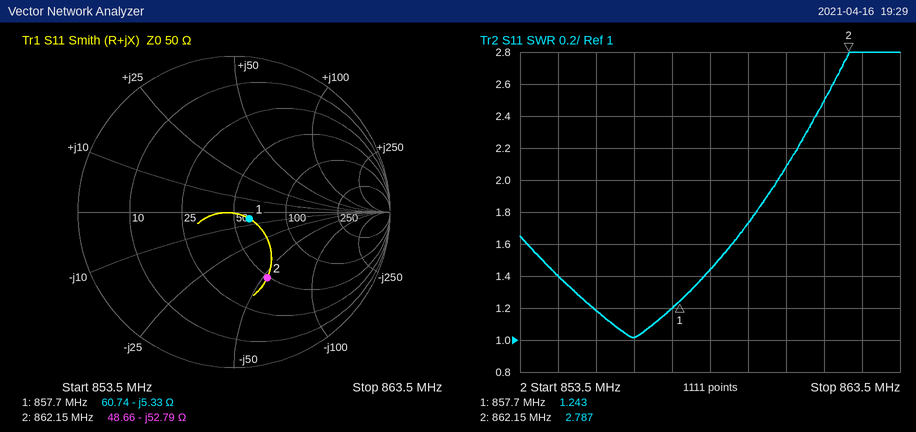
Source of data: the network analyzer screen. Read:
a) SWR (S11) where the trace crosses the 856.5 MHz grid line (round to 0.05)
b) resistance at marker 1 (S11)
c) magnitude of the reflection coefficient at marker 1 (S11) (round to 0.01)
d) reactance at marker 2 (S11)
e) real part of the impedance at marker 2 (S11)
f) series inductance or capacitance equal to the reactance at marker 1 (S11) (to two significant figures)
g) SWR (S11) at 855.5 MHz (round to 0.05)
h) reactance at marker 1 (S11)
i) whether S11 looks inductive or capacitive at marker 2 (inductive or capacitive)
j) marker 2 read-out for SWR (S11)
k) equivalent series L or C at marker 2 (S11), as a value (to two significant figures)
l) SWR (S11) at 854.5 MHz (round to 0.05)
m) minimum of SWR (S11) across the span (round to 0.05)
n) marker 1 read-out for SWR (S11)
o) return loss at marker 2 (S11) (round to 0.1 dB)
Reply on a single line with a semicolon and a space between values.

1.00; 60.74 Ω; 0.11; -52.79 Ω; 48.66 Ω; 35 pF; 1.20; -5.33 Ω; capacitive; 2.787; 3.5 pF; 1.40; 1.00; 1.243; 6.5 dB
